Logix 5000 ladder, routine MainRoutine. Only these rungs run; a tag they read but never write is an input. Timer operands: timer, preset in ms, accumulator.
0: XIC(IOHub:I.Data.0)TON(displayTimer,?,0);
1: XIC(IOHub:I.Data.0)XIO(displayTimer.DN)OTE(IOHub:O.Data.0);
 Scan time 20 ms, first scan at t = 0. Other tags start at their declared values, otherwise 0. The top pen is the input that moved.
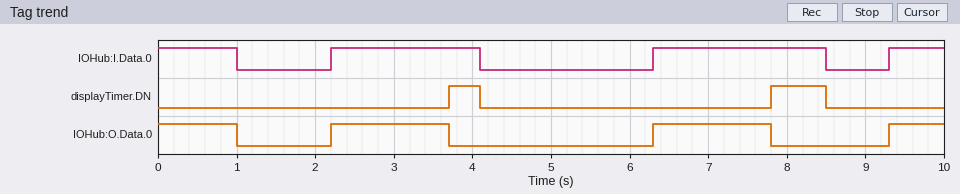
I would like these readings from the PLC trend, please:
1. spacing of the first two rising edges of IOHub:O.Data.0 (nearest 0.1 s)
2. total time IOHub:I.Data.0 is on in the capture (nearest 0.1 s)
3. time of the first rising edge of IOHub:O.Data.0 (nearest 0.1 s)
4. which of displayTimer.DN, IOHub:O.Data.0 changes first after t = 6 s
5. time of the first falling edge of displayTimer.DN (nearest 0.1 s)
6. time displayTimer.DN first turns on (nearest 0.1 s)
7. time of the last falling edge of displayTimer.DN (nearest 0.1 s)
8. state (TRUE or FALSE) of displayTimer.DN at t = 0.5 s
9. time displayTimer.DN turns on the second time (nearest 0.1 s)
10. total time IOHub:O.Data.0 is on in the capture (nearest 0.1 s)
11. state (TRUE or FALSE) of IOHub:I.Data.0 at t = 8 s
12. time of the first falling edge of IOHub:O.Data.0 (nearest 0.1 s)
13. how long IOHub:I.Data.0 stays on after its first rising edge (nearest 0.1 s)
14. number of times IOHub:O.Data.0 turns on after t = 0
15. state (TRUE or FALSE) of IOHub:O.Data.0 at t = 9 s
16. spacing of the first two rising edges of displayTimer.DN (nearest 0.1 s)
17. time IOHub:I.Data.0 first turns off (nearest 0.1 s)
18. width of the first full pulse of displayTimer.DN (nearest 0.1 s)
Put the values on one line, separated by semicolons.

4.1 s; 5.8 s; 2.2 s; IOHub:O.Data.0; 4.1 s; 3.7 s; 8.5 s; FALSE; 7.8 s; 4.7 s; TRUE; 1.0 s; 1.9 s; 3; FALSE; 4.1 s; 1.0 s; 0.4 s
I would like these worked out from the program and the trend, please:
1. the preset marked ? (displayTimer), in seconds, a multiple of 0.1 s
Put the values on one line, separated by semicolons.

1.5 s
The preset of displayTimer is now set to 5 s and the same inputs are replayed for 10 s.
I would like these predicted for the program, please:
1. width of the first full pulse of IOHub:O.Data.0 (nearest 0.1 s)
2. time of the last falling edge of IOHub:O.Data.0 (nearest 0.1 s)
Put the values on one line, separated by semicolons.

1.9 s; 8.5 s
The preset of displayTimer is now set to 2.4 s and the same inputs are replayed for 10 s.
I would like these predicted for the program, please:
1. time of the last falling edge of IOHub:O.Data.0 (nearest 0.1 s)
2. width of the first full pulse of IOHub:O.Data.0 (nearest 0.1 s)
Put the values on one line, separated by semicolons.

8.5 s; 1.9 s
